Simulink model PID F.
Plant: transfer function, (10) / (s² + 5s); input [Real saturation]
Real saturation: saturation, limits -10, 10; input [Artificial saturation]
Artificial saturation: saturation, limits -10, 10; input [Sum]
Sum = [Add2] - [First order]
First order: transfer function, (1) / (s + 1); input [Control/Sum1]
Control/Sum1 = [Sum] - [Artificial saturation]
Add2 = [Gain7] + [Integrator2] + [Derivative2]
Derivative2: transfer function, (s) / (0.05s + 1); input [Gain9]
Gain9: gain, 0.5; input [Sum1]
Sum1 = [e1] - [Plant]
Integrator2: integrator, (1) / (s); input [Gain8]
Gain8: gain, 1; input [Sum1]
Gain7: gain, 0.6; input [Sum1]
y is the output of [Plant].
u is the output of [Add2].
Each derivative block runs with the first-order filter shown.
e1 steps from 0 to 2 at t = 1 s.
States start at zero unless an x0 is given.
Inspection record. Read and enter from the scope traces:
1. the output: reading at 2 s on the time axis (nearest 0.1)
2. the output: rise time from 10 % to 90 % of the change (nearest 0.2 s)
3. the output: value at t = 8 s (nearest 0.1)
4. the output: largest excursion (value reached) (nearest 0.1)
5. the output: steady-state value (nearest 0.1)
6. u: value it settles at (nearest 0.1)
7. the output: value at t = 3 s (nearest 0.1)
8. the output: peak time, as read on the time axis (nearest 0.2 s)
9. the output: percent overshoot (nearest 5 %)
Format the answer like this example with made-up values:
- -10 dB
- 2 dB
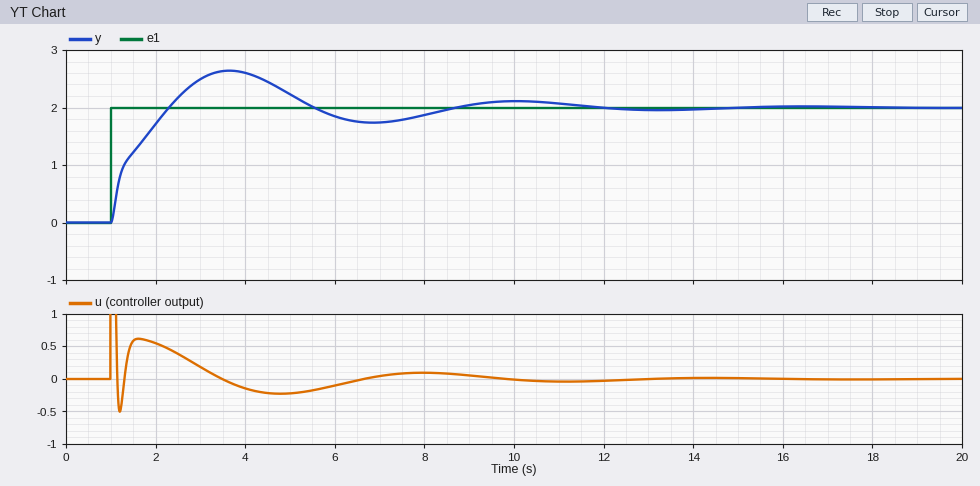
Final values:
- 1.7
- 1.0 s
- 1.9
- 2.6
- 2.0
- 0.0
- 2.5
- 3.6 s
- 30 %
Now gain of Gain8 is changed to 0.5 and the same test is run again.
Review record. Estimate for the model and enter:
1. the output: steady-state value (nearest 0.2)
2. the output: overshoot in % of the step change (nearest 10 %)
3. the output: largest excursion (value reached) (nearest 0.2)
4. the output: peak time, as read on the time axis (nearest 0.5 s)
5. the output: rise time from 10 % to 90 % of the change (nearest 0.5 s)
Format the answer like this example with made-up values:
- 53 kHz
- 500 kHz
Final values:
- 2.0
- 20 %
- 2.4
- 4.5 s
- 1.5 s
